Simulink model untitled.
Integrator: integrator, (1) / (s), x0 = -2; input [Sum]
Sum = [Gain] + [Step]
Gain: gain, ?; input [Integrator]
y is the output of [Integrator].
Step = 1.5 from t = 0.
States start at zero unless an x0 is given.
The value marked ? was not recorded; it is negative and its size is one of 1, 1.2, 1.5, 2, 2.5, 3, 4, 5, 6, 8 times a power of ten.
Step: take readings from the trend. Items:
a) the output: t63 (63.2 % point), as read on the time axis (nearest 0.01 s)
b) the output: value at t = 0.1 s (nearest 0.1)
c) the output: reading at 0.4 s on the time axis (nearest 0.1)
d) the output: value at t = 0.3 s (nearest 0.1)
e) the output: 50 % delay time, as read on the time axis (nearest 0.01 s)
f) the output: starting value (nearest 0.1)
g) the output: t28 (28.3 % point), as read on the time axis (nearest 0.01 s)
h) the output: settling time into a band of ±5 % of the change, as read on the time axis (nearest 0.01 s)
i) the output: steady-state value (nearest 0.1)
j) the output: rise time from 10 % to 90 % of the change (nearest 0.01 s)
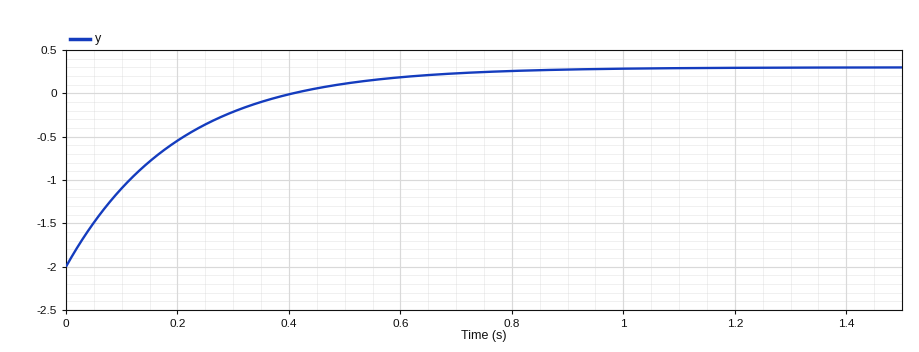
0.20 s
-1.1
0.0
-0.2
0.14 s
-2.0
0.07 s
0.60 s
0.3
0.44 s
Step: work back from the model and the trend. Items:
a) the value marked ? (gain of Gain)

-5
